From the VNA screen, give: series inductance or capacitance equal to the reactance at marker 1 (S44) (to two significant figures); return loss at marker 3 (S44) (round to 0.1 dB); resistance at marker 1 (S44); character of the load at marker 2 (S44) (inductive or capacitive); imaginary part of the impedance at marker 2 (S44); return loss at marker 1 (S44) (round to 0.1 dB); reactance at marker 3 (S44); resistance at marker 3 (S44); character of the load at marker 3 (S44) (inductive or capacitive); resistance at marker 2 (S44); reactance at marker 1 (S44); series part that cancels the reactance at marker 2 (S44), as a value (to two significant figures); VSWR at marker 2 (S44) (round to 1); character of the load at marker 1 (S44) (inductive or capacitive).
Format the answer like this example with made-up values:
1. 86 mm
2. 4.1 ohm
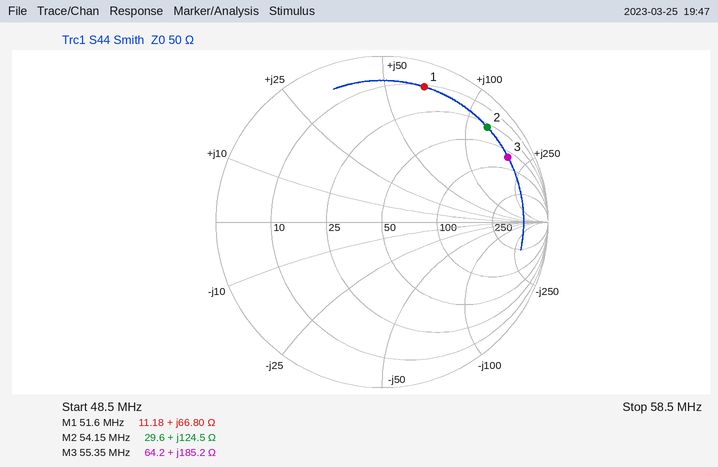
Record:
1. 210 nH
2. 1.4 dB
3. 11.18 Ω
4. inductive
5. +124.5 Ω
6. 1.4 dB
7. +185.2 Ω
8. 64.2 Ω
9. inductive
10. 29.6 Ω
11. +66.80 Ω
12. 24 pF
13. 13
14. inductive
